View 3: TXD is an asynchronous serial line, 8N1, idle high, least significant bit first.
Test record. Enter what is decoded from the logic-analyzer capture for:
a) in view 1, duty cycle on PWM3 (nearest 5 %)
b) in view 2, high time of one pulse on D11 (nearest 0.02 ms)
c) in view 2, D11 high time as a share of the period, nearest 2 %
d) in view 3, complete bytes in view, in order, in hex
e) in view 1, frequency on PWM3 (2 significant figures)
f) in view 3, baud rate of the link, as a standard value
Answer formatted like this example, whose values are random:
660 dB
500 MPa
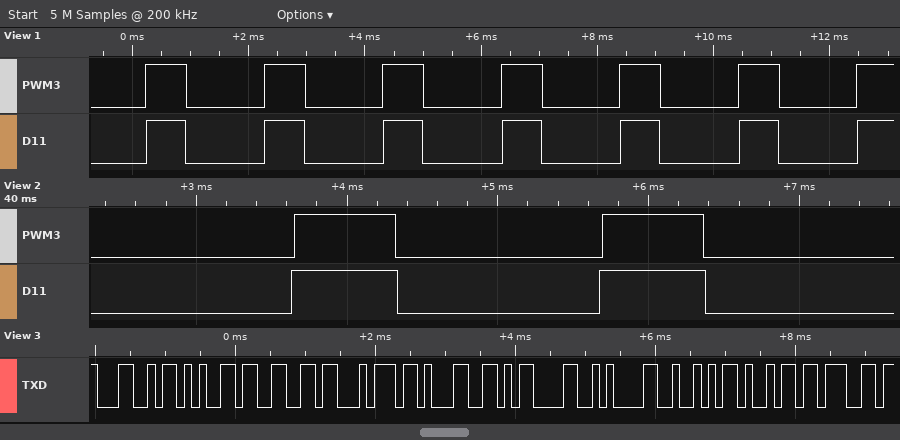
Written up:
35 %
0.70 ms
34 %
0x4C 0x65 0x66 0x74 0x31 0x0D 0x0A 0x52 0x69 0x67
490 Hz
9600 baud
